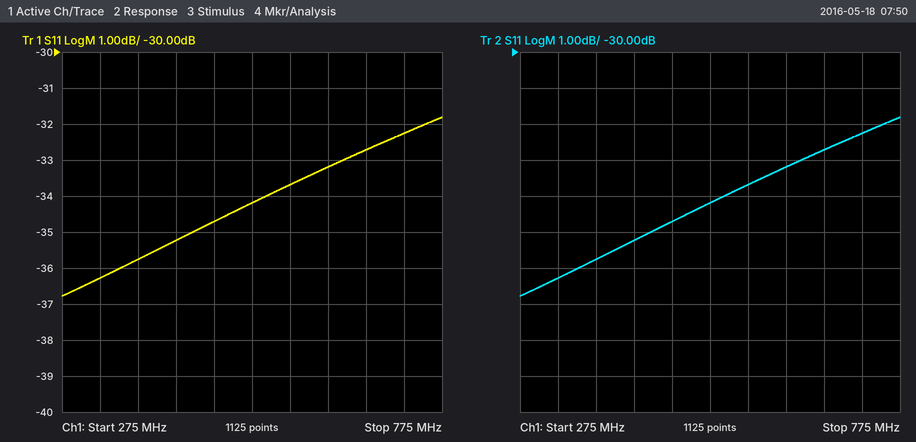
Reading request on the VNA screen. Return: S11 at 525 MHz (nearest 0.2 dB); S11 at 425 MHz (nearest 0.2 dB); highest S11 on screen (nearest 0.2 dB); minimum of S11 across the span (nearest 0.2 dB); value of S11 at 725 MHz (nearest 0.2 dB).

-34.2 dB
-35.2 dB
-31.8 dB
-36.8 dB
-32.2 dB
